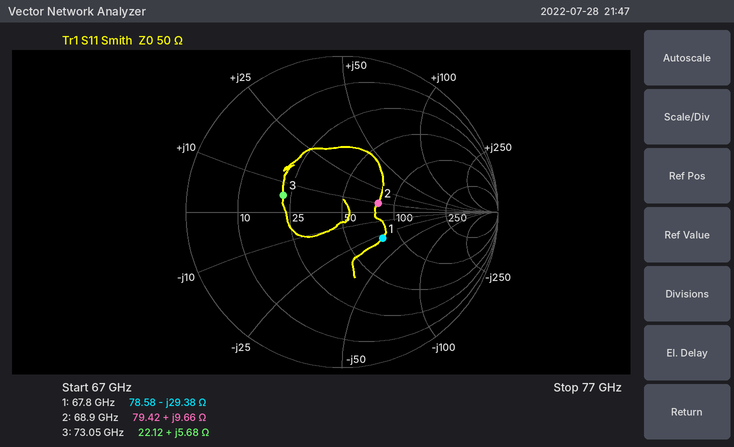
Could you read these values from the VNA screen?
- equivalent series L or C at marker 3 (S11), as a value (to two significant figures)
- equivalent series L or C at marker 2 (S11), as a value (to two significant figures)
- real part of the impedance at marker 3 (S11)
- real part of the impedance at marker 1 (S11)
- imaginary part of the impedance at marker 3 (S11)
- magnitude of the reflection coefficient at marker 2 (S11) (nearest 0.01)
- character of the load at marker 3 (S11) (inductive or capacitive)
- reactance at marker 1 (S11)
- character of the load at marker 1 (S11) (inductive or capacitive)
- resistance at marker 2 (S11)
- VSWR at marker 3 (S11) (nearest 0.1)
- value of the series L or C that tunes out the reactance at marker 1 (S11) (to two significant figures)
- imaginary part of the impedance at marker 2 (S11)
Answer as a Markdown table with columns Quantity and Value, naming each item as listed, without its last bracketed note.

| Quantity | Value |
|---|---|
| equivalent series L or C at marker 3 (S11), as a value | 12 pH |
| equivalent series L or C at marker 2 (S11), as a value | 22 pH |
| real part of the impedance at marker 3 | 22.12 Ω |
| real part of the impedance at marker 1 | 78.58 Ω |
| imaginary part of the impedance at marker 3 | +5.68 Ω |
| magnitude of the reflection coefficient at marker 2 (S11) | 0.24 |
| character of the load at marker 3 (S11) | inductive |
| reactance at marker 1 | -29.38 Ω |
| character of the load at marker 1 (S11) | capacitive |
| resistance at marker 2 | 79.42 Ω |
| VSWR at marker 3 (S11) | 2.3 |
| value of the series L or C that tunes out the reactance at marker 1 (S11) | 69 pH |
| imaginary part of the impedance at marker 2 | +9.66 Ω |
